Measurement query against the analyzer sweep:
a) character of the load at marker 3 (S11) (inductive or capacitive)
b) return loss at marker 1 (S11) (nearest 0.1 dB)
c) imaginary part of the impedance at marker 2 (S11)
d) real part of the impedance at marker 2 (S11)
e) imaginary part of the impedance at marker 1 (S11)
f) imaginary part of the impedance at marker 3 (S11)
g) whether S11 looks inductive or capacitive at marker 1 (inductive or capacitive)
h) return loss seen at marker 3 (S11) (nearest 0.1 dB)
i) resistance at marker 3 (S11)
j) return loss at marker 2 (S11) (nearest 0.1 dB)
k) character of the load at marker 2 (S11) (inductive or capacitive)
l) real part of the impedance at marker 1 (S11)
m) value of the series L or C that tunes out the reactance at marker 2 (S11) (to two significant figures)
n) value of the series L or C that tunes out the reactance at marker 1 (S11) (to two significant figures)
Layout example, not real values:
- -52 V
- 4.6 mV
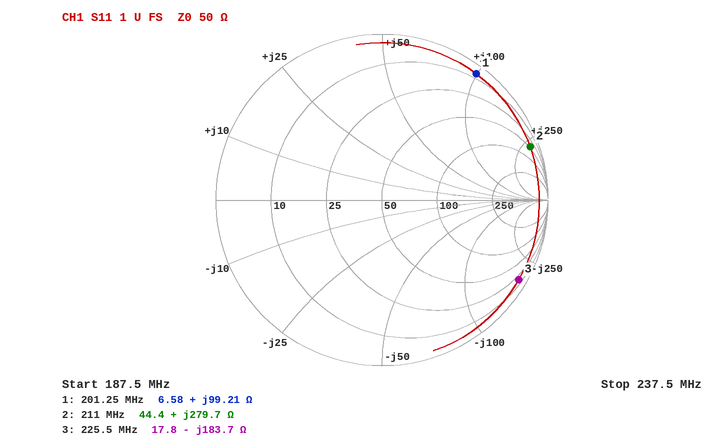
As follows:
- capacitive
- 0.5 dB
- +279.7 Ω
- 44.4 Ω
- +99.21 Ω
- -183.7 Ω
- inductive
- 0.4 dB
- 17.8 Ω
- 0.5 dB
- inductive
- 6.58 Ω
- 2.7 pF
- 8.0 pF
